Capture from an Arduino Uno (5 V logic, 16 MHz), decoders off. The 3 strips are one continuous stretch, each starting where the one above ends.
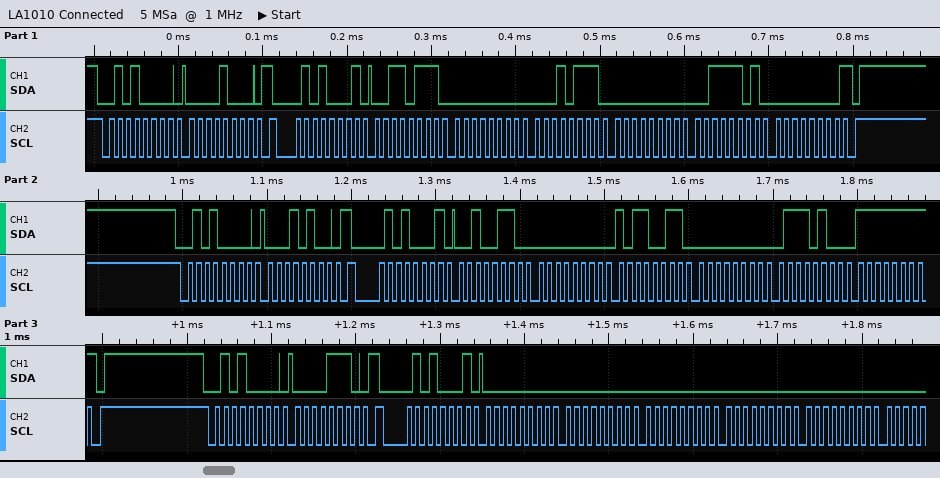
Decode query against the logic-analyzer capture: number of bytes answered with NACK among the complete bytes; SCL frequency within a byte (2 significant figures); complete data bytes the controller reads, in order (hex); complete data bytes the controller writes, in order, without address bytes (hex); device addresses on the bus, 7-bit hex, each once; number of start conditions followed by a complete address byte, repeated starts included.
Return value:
2
100 kHz
37 00 17 00 3D 00 26 00 B3 00 74 FF 00 00 00 00 00
08 14 0E
0x28
6
